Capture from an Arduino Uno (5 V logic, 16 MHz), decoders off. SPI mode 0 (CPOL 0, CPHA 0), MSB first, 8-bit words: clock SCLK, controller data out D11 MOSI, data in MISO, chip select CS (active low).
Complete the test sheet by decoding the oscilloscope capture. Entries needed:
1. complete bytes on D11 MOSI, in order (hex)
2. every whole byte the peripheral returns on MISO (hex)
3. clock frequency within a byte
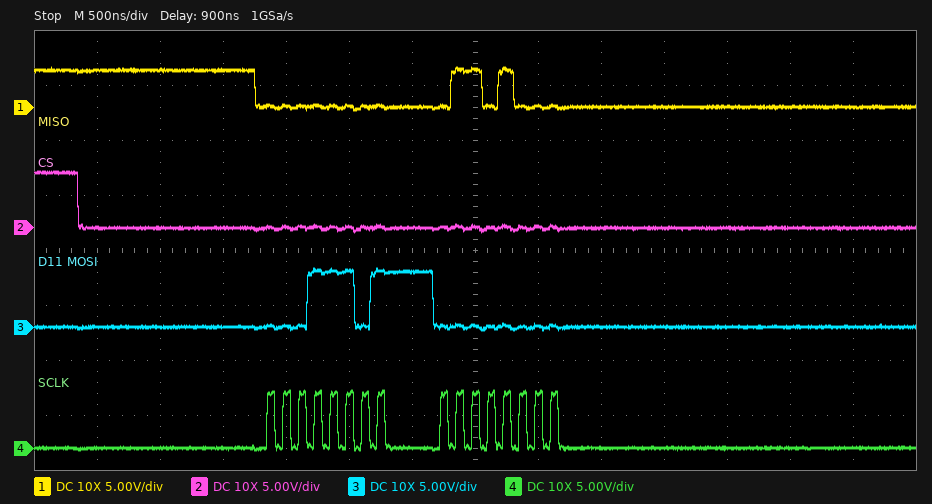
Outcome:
1D 00
00 68
8 MHz
